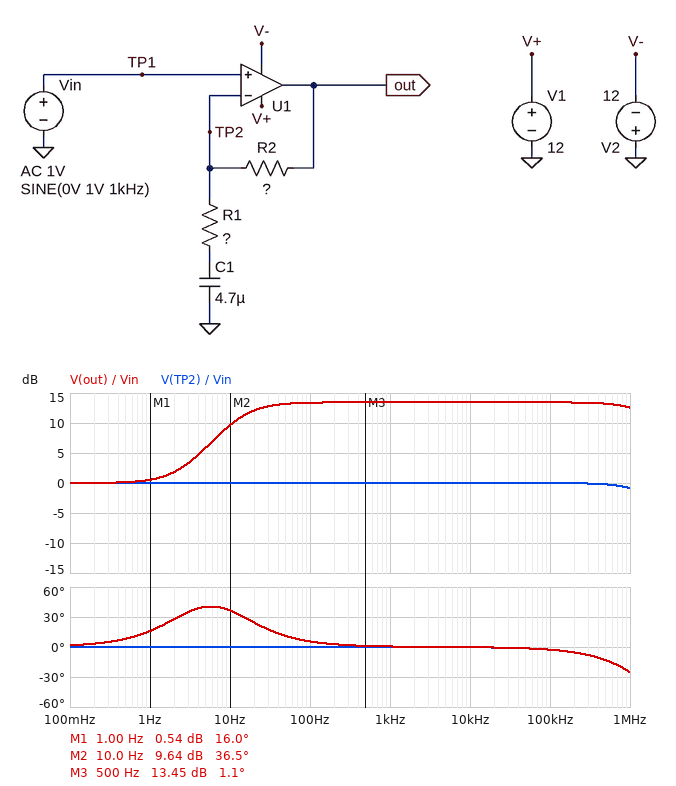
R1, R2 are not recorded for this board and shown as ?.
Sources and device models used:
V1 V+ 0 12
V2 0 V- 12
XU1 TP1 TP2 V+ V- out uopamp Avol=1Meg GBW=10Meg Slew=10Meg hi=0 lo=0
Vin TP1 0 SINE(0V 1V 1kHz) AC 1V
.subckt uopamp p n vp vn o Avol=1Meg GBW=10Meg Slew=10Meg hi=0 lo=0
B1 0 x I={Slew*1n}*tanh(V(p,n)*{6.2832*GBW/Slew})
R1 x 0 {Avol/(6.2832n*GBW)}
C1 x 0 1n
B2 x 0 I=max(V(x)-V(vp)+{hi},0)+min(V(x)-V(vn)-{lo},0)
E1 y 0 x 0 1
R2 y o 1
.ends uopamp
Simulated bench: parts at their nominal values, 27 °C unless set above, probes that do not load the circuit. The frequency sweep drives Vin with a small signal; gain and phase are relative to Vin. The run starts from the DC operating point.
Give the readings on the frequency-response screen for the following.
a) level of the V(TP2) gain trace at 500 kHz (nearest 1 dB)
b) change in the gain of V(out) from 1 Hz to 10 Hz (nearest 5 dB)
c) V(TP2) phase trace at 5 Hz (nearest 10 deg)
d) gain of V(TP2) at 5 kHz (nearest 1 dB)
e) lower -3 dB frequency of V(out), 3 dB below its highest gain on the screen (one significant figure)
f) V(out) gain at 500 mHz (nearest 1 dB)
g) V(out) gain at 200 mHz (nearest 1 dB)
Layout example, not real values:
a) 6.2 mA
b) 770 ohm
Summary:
a) 0 dB
b) 10 dB
c) 0 deg
d) 0 dB
e) 10 Hz
f) 0 dB
g) 0 dB
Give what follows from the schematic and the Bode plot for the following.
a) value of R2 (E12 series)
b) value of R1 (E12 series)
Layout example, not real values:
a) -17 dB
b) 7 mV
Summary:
a) 10 kΩ
b) 2.7 kΩ
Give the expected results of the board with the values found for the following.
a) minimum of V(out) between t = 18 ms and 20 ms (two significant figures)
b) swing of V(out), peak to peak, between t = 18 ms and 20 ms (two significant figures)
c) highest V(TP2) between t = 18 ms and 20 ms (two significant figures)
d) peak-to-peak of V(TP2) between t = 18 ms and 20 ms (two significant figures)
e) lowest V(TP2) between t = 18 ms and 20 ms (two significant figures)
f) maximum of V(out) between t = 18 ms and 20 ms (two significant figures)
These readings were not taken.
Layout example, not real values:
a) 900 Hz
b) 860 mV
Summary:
a) -4.7 V
b) 9.4 V
c) 1.0 V
d) 2.0 V
e) -1.0 V
f) 4.7 V
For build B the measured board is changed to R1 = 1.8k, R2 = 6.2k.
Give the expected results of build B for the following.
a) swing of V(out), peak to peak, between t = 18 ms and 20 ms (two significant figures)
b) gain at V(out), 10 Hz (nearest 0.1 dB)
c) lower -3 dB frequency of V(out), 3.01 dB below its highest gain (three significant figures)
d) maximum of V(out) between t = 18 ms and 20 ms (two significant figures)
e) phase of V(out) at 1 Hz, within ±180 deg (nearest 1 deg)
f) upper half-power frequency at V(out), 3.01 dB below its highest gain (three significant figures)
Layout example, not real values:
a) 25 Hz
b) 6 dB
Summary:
a) 8.9 V
b) 7.1 dB
c) 17.8 Hz
d) 4.4 V
e) 10 deg
f) 2.25 MHz
